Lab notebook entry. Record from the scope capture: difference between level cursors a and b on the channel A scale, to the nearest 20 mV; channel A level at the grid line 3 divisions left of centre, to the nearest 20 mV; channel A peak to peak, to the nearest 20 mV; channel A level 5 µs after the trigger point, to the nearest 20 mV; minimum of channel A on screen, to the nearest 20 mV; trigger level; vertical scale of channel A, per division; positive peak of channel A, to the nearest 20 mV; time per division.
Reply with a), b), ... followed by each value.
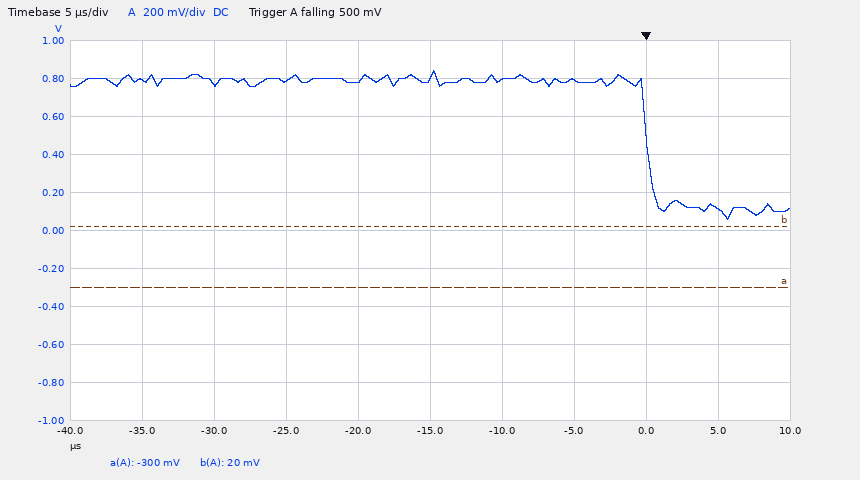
a) 320 mV
b) 780 mV
c) 780 mV
d) 120 mV
e) 60 mV
f) 500 mV
g) 200 mV
h) 840 mV
i) 5 µs
